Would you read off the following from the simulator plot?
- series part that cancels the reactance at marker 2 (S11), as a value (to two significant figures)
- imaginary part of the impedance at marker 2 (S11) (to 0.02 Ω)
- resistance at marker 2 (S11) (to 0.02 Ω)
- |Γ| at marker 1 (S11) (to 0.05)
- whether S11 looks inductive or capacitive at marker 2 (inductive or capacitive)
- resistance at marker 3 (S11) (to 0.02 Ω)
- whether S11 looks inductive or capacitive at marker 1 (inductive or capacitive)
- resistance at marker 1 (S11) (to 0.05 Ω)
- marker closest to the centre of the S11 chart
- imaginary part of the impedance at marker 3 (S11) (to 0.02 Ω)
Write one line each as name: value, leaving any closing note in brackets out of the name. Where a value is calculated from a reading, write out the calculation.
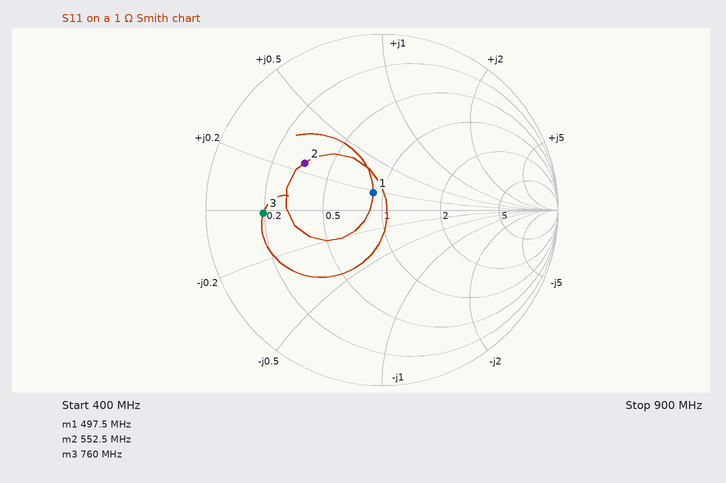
series part that cancels the reactance at marker 2 (S11), as a value: C = 1/(2π × 552.5 MHz × 0.24 Ω) ≈ 1.2 nF
imaginary part of the impedance at marker 2 (S11): +0.24 Ω
resistance at marker 2 (S11): 0.34 Ω
|Γ| at marker 1 (S11): 0.10
whether S11 looks inductive or capacitive at marker 2: inductive
resistance at marker 3 (S11): 0.20 Ω
whether S11 looks inductive or capacitive at marker 1: inductive
resistance at marker 1 (S11): 0.90 Ω
marker closest to the centre of the S11 chart: marker 1
imaginary part of the impedance at marker 3 (S11): -0.02 Ω
